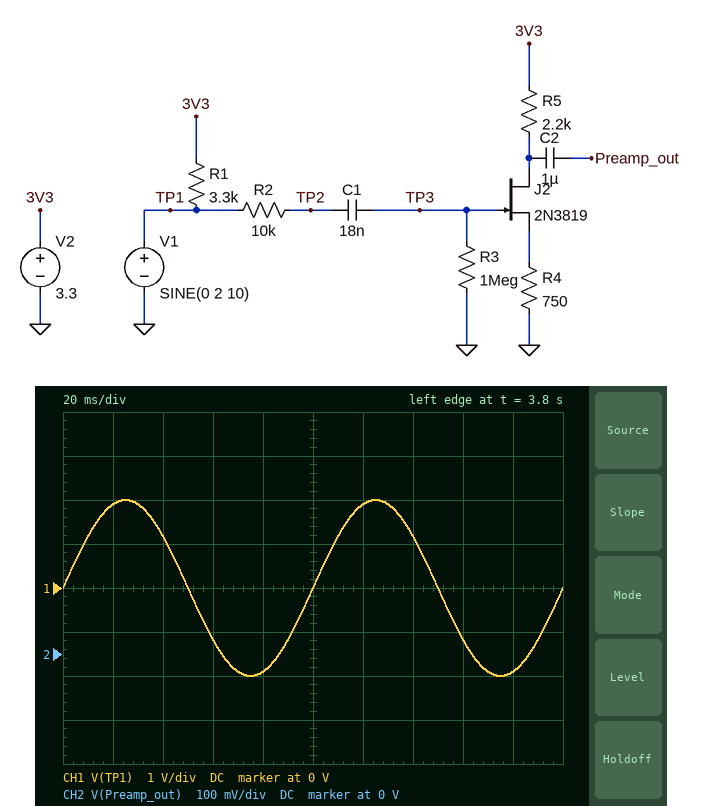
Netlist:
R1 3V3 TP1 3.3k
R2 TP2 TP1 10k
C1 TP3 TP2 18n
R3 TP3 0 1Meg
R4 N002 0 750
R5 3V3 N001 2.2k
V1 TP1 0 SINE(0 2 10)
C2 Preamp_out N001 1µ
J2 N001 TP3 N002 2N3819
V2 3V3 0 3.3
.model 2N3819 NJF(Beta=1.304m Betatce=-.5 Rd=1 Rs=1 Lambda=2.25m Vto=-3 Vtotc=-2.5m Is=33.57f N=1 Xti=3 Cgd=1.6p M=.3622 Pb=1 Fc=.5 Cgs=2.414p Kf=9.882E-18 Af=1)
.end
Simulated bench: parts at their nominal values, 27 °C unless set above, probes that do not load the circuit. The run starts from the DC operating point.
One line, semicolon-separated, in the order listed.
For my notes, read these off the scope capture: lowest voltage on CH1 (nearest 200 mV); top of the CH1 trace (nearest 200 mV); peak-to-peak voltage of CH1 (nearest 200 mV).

-2.0 V; 2.0 V; 4.0 V
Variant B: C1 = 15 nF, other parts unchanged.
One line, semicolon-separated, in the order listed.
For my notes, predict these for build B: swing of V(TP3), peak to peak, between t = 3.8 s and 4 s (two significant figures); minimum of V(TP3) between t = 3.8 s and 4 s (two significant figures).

2.6 V; -1.4 V
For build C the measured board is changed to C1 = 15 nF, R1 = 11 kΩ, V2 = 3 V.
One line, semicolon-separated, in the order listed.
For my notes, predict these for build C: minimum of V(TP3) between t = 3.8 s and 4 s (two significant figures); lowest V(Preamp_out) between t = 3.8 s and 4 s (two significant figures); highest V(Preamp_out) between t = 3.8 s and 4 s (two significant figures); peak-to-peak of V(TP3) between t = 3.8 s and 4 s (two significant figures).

-1.4 V; 850 mV; 1.1 V; 2.5 V
